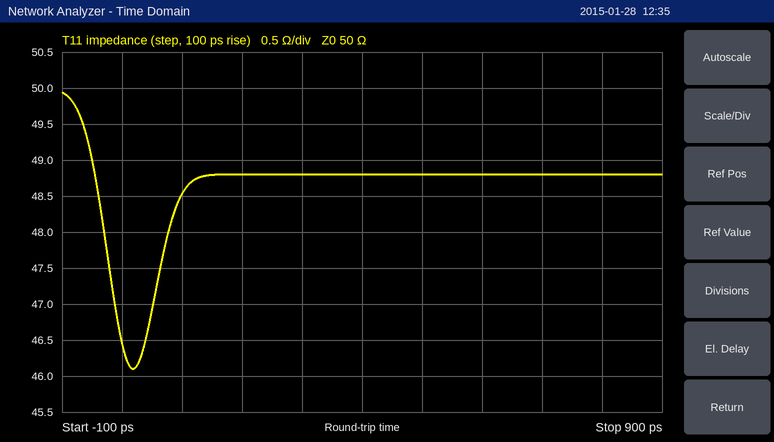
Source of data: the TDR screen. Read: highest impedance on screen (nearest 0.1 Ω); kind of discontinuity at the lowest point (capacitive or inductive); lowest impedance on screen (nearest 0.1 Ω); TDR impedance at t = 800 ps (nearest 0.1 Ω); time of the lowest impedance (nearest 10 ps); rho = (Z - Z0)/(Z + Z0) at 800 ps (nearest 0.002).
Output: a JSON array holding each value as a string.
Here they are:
["49.9 Ω", "capacitive", "46.1 Ω", "48.8 Ω", "20 ps", "-0.012"]
